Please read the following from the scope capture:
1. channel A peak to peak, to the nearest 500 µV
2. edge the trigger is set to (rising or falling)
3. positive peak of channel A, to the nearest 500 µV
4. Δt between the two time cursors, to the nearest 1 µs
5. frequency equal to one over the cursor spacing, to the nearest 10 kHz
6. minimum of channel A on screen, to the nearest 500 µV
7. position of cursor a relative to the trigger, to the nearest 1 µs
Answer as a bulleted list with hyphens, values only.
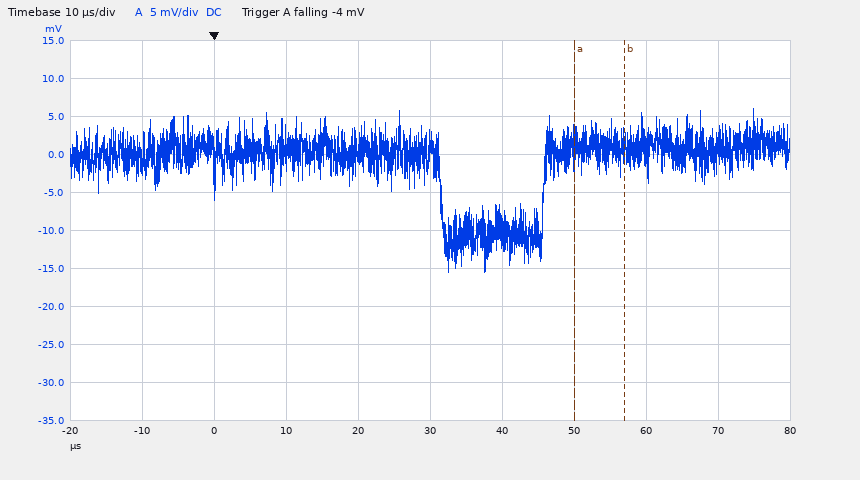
- 21.5 mV
- falling
- 6.0 mV
- 7 µs
- 140 kHz
- -15.5 mV
- +50 µs
